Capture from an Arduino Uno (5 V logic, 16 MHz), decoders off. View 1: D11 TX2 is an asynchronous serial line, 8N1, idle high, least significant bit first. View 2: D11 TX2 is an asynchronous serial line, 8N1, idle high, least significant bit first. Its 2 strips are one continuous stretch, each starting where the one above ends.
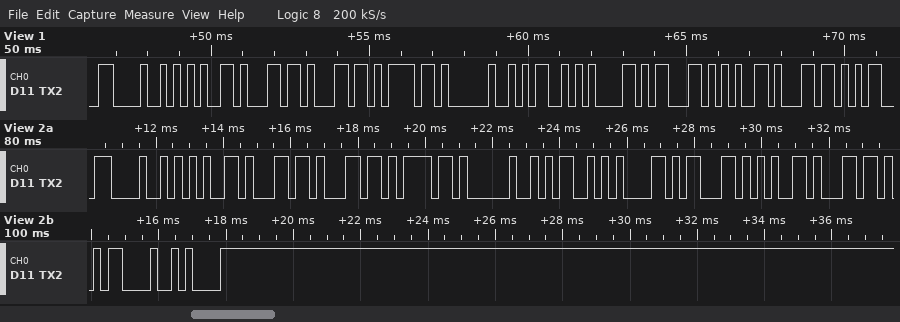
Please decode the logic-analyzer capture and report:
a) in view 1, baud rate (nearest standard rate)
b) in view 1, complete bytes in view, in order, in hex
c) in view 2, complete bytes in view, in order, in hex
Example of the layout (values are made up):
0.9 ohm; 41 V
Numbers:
4800 baud; 48 65 6C 6C 6F 20 4D 61 63 65 6C; 48 65 6C 6C 6F 20 4D 61 63 65 6C 0D 0A
